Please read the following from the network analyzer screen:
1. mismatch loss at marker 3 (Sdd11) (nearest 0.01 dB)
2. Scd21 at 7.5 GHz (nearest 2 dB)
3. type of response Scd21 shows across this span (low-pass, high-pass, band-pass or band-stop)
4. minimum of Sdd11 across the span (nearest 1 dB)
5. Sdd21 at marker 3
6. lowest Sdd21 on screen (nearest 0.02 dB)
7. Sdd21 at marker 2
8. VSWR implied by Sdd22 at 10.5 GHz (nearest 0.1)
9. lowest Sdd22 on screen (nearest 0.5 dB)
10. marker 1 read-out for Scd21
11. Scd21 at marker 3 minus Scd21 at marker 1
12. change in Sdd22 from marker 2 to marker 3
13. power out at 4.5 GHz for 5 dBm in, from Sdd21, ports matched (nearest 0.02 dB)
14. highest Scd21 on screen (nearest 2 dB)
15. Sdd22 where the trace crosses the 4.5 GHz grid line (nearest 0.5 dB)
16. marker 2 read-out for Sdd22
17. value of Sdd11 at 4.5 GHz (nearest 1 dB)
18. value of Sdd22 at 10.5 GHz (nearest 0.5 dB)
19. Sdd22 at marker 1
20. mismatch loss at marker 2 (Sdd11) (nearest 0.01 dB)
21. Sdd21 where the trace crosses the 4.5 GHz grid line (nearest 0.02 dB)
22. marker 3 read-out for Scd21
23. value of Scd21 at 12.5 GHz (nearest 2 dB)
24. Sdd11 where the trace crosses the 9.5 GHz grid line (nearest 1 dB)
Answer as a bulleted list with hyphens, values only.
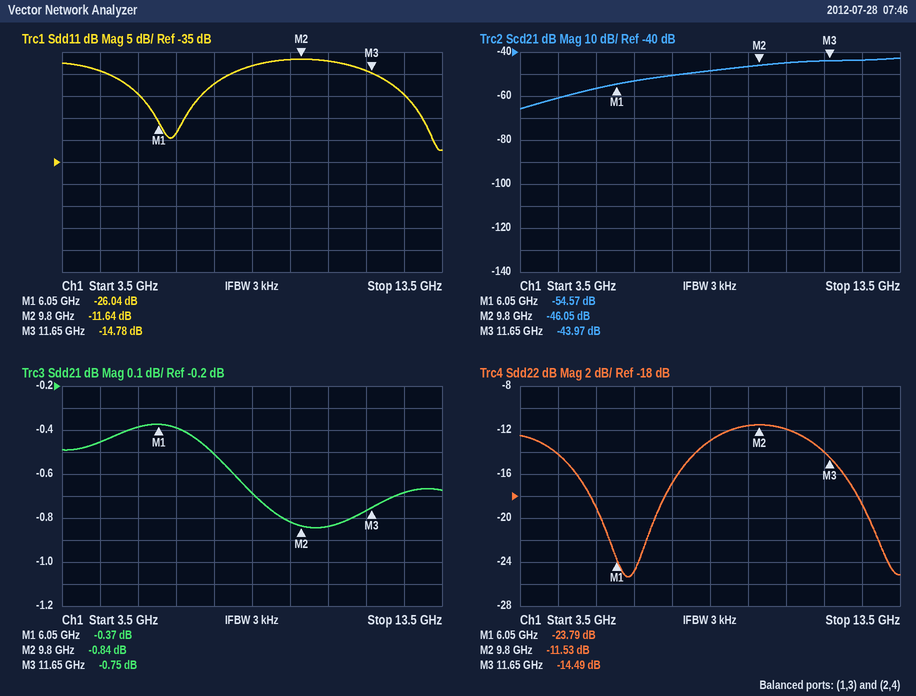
- 0.15 dB
- -50 dB
- high-pass
- -32 dB
- -0.75 dB
- -0.84 dB
- -0.84 dB
- 1.7
- -25.5 dB
- -54.57 dB
- 10.60 dB
- -2.96 dB
- 4.54 dBm
- -42 dB
- -14.0 dB
- -11.53 dB
- -14 dB
- -12.0 dB
- -23.79 dB
- 0.31 dB
- -0.46 dB
- -43.97 dB
- -44 dB
- -12 dB
